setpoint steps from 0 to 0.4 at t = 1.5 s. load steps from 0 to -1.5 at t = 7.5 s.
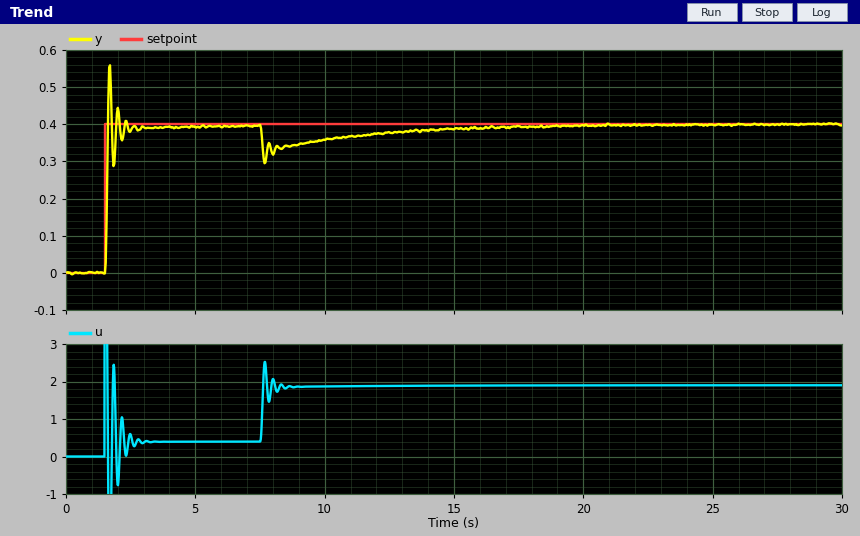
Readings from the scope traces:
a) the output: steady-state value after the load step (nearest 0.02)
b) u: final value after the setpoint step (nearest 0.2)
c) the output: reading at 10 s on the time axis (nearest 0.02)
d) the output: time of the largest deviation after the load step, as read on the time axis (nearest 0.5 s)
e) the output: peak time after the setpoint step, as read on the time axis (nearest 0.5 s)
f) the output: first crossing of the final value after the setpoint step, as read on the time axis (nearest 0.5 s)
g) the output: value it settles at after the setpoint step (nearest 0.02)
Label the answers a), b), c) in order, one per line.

a) 0.40
b) 0.4
c) 0.36
d) 7.5 s
e) 1.5 s
f) 1.5 s
g) 0.40
